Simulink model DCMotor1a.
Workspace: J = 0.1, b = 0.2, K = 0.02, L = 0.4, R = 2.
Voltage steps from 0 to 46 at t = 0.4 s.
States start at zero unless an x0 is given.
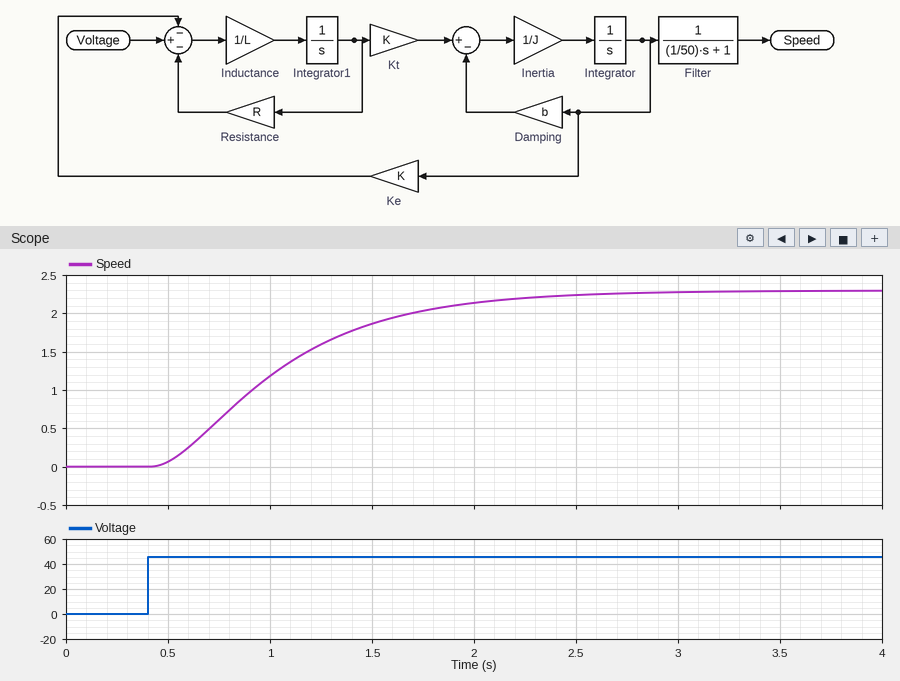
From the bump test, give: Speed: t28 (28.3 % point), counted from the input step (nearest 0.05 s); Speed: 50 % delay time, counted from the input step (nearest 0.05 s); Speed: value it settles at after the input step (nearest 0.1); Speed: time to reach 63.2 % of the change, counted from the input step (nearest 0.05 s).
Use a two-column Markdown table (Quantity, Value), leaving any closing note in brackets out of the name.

| Quantity | Value |
|---|---|
| Speed: t28 (28.3 % point), counted from the input step | 0.35 s |
| Speed: 50 % delay time, counted from the input step | 0.60 s |
| Speed: value it settles at after the input step | 2.3 |
| Speed: time to reach 63.2 % of the change, counted from the input step | 0.75 s |
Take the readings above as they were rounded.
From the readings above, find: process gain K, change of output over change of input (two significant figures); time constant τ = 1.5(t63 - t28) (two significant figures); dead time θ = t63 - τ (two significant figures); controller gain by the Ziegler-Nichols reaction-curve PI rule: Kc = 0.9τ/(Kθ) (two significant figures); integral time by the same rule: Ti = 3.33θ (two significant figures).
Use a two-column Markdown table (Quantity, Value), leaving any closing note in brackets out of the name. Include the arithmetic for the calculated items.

| Quantity | Value |
|---|---|
| process gain K, change of output over change of input | (2.3 - 0) / 46 = 0.050 |
| time constant τ = 1.5(t63 - t28) | 1.5 × (0.75 - 0.35) = 0.60 s |
| dead time θ = t63 - τ | 0.75 - 0.6 = 0.15 s |
| controller gain by the Ziegler-Nichols reaction-curve PI rule: Kc = 0.9τ/(Kθ) | 0.9 × 0.6 / (0.05 × 0.15) = 72 |
| integral time by the same rule: Ti = 3.33θ | 3.33 × 0.15 = 0.50 s |
